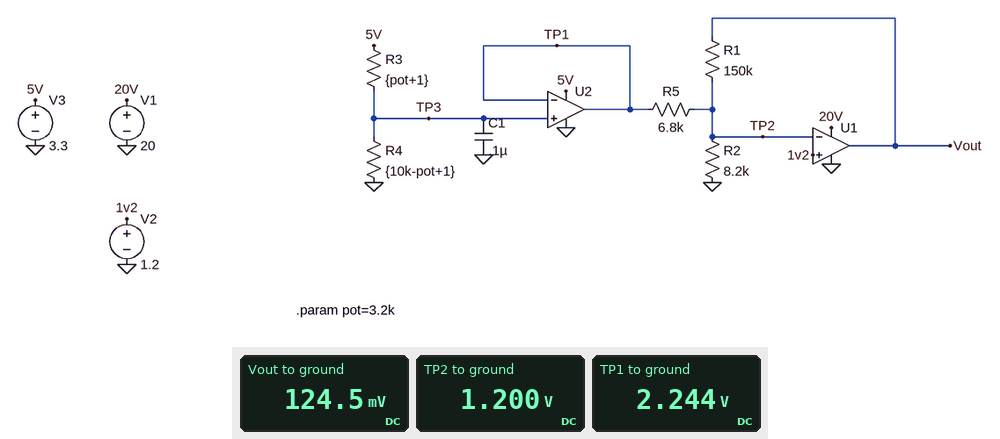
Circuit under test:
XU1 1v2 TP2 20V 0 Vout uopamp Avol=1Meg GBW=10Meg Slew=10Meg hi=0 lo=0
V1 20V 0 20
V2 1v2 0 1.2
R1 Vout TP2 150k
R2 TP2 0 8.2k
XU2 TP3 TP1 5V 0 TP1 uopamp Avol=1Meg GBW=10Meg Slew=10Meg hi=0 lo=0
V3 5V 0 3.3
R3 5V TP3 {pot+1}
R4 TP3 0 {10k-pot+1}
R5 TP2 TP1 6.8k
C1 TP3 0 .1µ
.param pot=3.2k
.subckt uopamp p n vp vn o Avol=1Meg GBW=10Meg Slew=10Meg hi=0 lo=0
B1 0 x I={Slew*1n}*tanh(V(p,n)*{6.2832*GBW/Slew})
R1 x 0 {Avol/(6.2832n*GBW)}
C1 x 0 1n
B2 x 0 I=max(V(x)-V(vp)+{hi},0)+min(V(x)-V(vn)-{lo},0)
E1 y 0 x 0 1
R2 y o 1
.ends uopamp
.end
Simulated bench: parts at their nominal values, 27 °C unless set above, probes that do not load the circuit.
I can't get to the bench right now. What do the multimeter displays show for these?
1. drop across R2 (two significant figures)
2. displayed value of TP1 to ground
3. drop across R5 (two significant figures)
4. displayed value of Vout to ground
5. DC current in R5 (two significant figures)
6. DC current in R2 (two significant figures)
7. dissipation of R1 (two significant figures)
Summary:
1.2 V
2.244 V
1.0 V
124.5 mV
150 µA
150 µA
7.7 µW
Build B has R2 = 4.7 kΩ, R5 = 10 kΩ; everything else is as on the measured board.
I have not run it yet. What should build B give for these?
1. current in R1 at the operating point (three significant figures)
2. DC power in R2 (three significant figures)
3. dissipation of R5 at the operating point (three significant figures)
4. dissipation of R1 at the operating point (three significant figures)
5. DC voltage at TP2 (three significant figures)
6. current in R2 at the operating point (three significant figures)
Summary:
126 µA
267 µW
126 µW
2.38 mW
1.12 V
238 µA
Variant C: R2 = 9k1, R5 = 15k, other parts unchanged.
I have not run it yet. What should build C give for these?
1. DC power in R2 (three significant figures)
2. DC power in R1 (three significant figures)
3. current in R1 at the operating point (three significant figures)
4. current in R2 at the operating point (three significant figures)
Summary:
158 µW
582 µW
62.3 µA
132 µA
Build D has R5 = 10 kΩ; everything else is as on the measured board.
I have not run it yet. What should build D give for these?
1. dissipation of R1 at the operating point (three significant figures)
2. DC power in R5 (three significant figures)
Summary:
264 µW
109 µW
